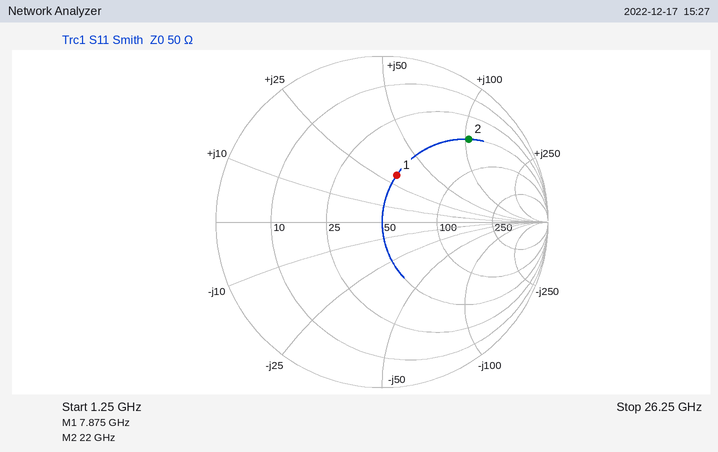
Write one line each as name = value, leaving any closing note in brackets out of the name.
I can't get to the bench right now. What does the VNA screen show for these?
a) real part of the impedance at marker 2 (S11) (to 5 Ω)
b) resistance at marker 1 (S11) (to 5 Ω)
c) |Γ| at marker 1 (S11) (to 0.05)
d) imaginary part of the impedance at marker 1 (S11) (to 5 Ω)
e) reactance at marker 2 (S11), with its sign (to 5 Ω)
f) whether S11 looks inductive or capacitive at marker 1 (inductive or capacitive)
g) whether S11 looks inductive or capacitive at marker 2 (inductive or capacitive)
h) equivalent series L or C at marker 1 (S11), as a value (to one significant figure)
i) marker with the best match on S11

real part of the impedance at marker 2 (S11) = 50 Ω
resistance at marker 1 (S11) = 50 Ω
|Γ| at marker 1 (S11) = 0.30
imaginary part of the impedance at marker 1 (S11) = +30 Ω
reactance at marker 2 (S11), with its sign = +105 Ω
whether S11 looks inductive or capacitive at marker 1 = inductive
whether S11 looks inductive or capacitive at marker 2 = inductive
equivalent series L or C at marker 1 (S11), as a value = 600 pH
marker with the best match on S11 = marker 1
